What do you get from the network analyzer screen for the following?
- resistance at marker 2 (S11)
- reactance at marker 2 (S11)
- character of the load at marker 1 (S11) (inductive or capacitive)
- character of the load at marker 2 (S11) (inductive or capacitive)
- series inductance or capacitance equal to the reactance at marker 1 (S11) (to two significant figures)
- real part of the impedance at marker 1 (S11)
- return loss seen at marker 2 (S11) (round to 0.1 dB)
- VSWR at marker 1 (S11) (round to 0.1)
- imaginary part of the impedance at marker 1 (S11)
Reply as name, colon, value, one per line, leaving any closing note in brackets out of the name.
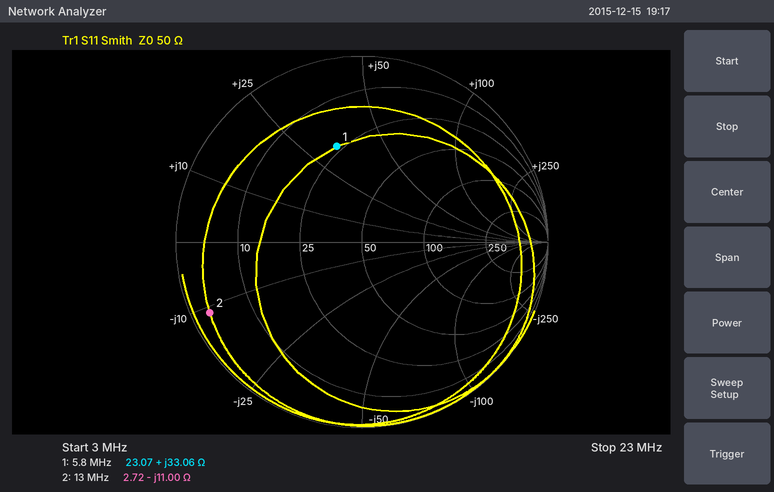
resistance at marker 2: 2.72 Ω
reactance at marker 2: -11.00 Ω
character of the load at marker 1 (S11): inductive
character of the load at marker 2 (S11): capacitive
series inductance or capacitance equal to the reactance at marker 1 (S11): 910 nH
real part of the impedance at marker 1: 23.07 Ω
return loss seen at marker 2 (S11): 0.9 dB
VSWR at marker 1 (S11): 3.3
imaginary part of the impedance at marker 1: +33.06 Ω
